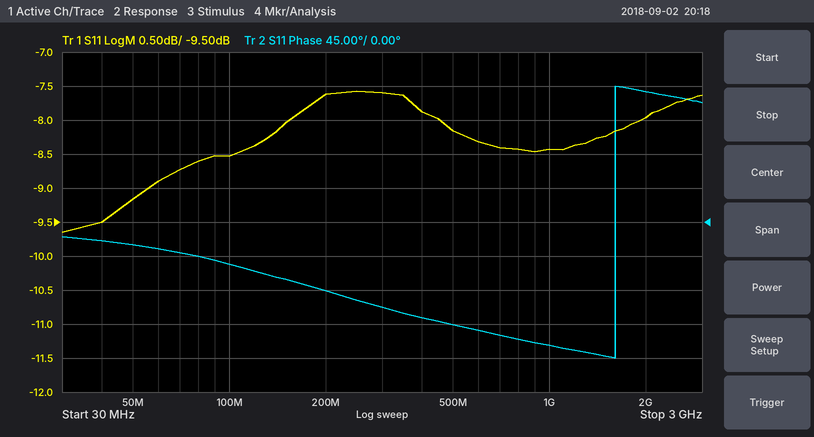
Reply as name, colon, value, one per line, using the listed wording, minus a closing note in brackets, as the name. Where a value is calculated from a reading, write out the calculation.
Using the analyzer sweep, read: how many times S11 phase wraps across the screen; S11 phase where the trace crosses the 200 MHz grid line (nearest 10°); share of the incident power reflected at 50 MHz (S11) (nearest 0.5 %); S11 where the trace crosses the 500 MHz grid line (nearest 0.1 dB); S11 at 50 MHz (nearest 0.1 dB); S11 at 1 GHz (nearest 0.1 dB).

how many times S11 phase wraps across the screen: 1
S11 phase where the trace crosses the 200 MHz grid line: -90°
share of the incident power reflected at 50 MHz (S11): 10^(-9.2/10) ≈ 12.0 %
S11 where the trace crosses the 500 MHz grid line: -8.2 dB
S11 at 50 MHz: -9.2 dB
S11 at 1 GHz: -8.4 dB
